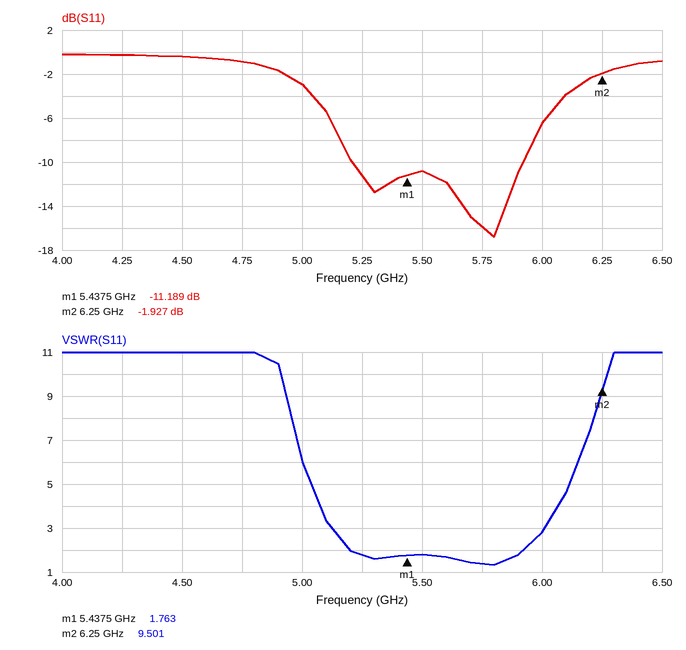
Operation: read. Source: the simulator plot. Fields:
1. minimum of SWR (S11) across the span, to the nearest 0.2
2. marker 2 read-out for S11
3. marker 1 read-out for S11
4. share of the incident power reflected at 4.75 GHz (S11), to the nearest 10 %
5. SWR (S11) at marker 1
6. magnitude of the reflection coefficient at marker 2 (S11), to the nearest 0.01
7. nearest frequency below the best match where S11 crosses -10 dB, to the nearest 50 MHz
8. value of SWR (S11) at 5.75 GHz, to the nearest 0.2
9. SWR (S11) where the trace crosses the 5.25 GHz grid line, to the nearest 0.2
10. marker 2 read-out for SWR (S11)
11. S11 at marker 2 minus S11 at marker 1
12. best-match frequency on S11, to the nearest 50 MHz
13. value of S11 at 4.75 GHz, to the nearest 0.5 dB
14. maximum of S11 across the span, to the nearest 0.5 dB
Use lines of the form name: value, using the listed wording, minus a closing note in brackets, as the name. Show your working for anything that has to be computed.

minimum of SWR (S11) across the span, to the nearest 0.2: 1.4
marker 2 read-out for S11: -1.927 dB
marker 1 read-out for S11: -11.189 dB
share of the incident power reflected at 4.75 GHz (S11), to the nearest 10 %: 10^(-1/10) ≈ 79.4 %, so 80 % to the nearest 10 %
SWR (S11) at marker 1: 1.763
magnitude of the reflection coefficient at marker 2 (S11), to the nearest 0.01: 10^(-1.927/20) ≈ 0.80
nearest frequency below the best match where S11 crosses -10 dB, to the nearest 50 MHz: 5.20 GHz
value of SWR (S11) at 5.75 GHz, to the nearest 0.2: 1.4
SWR (S11) where the trace crosses the 5.25 GHz grid line, to the nearest 0.2: 1.8
marker 2 read-out for SWR: 9.501
S11 at marker 2 minus S11 at marker 1: -1.927 − (-11.189) = 9.262 dB
best-match frequency on S11, to the nearest 50 MHz: 5.80 GHz
value of S11 at 4.75 GHz, to the nearest 0.5 dB: -1.0 dB
maximum of S11 across the span, to the nearest 0.5 dB: 0.0 dB
